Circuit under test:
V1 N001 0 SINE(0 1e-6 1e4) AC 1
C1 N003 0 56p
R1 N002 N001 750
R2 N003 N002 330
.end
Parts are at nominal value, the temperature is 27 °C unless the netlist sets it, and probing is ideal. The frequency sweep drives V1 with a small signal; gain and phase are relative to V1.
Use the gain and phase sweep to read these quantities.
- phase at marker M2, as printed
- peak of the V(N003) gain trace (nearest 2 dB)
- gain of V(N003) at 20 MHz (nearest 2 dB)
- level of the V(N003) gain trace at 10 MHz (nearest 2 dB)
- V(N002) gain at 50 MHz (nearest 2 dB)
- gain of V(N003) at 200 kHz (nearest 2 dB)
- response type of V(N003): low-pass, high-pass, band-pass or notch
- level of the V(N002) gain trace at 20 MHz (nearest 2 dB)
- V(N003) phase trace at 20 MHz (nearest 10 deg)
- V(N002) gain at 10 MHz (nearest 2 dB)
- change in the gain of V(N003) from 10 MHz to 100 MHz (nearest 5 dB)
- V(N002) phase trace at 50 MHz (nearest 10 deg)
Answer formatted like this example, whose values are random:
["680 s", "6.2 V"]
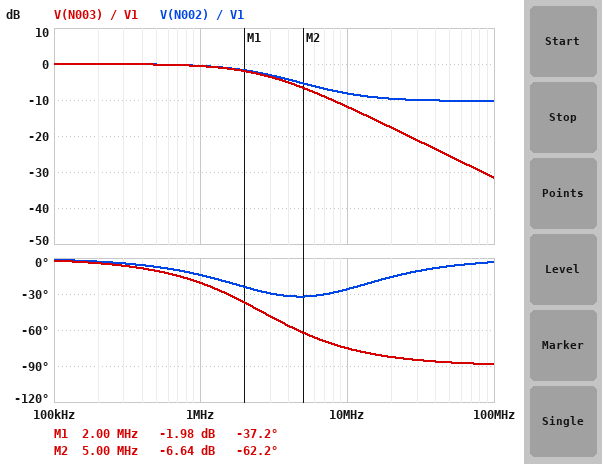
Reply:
["-62.2 deg", "0 dB", "-18 dB", "-12 dB", "-10 dB", "0 dB", "low-pass", "-10 dB", "-80 deg", "-8 dB", "-20 dB", "-10 deg"]
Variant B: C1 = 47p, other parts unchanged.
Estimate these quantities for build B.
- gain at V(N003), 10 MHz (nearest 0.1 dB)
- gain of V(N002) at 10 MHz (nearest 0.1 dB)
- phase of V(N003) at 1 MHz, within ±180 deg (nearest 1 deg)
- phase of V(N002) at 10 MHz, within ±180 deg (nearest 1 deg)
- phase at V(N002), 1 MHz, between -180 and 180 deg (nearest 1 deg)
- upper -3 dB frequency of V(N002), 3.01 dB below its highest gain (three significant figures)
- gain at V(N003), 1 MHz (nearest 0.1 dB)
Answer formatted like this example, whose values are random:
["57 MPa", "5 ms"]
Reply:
["-10.5 dB", "-7.6 dB", "-18 deg", "-28 deg", "-12 deg", "3.48 MHz", "-0.4 dB"]
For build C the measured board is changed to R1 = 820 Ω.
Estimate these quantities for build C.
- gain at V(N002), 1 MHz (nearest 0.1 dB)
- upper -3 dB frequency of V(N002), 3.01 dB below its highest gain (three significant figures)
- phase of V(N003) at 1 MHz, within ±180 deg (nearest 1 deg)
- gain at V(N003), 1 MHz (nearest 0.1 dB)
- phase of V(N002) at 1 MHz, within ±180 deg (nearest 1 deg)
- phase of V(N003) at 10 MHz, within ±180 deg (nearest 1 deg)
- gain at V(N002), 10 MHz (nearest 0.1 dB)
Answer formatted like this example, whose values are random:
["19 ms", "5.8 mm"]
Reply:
["-0.6 dB", "2.70 MHz", "-22 deg", "-0.7 dB", "-15 deg", "-76 deg", "-8.7 dB"]
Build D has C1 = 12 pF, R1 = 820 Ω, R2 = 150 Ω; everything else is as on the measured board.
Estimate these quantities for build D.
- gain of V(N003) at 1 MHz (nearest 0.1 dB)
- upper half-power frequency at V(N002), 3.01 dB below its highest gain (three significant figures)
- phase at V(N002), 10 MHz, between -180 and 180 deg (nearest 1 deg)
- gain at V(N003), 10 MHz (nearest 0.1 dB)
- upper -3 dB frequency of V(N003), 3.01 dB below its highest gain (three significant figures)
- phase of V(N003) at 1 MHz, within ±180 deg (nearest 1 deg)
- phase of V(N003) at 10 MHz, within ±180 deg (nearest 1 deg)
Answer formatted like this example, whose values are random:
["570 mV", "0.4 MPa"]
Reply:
["0 dB", "14.0 MHz", "-30 deg", "-1.9 dB", "13.7 MHz", "-4 deg", "-36 deg"]
